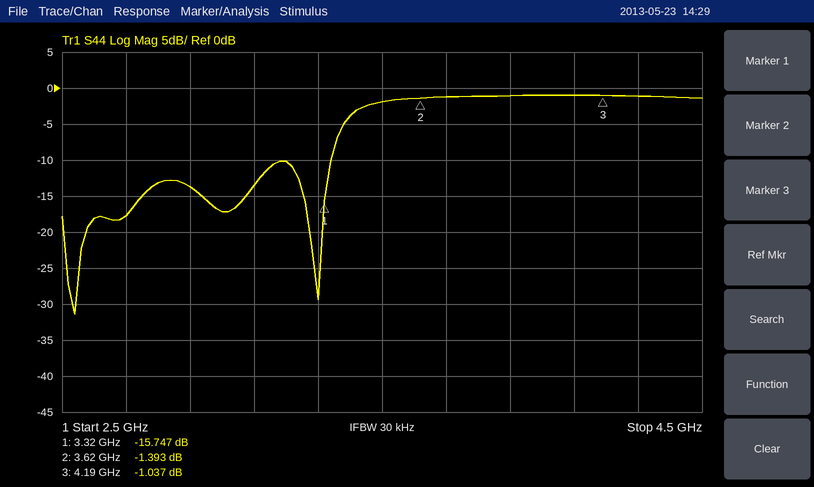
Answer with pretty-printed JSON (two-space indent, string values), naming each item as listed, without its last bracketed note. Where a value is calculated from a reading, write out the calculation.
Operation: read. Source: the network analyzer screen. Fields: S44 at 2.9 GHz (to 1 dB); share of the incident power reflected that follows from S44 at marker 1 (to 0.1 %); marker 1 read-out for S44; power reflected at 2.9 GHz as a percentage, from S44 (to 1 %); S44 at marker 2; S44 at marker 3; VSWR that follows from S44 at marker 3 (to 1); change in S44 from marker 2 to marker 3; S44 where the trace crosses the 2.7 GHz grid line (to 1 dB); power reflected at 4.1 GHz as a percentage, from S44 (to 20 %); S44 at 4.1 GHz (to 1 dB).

{
  "S44 at 2.9 GHz": "-14 dB",
  "share of the incident power reflected that follows from S44 at marker 1": "10^(-15.747/10) ≈ 2.7 %",
  "marker 1 read-out for S44": "-15.747 dB",
  "power reflected at 2.9 GHz as a percentage, from S44": "10^(-14/10) ≈ 4 %",
  "S44 at marker 2": "-1.393 dB",
  "S44 at marker 3": "-1.037 dB",
  "VSWR that follows from S44 at marker 3": "(1 + 0.8875)/(1 − 0.8875) ≈ 17",
  "change in S44 from marker 2 to marker 3": "-1.037 − (-1.393) = 0.356 dB",
  "S44 where the trace crosses the 2.7 GHz grid line": "-18 dB",
  "power reflected at 4.1 GHz as a percentage, from S44": "10^(-1/10) ≈ 79.4 %, so 80 % to the nearest 20 %",
  "S44 at 4.1 GHz": "-1 dB"
}
